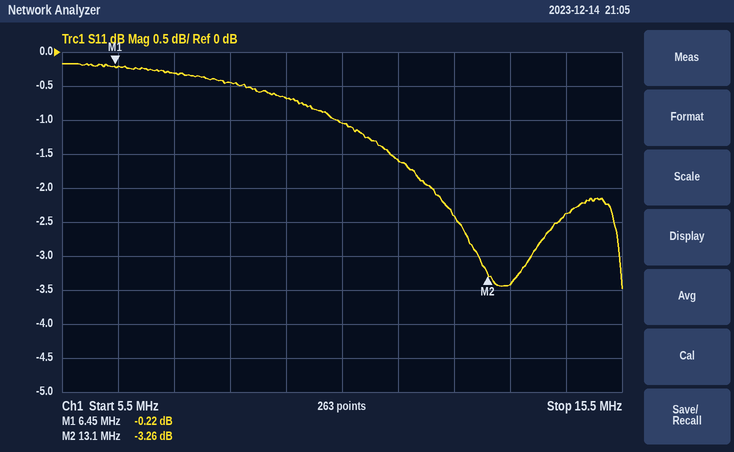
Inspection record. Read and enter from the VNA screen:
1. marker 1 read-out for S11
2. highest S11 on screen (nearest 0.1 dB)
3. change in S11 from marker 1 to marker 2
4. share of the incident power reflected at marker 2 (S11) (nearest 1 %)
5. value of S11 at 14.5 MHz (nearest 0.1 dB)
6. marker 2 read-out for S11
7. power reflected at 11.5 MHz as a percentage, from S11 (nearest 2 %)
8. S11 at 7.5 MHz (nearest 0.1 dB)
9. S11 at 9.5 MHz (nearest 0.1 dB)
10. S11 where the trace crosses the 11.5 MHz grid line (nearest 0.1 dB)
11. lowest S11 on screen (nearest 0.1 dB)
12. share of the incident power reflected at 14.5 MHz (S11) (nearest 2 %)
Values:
-0.22 dB
-0.2 dB
-3.04 dB
47 %
-2.4 dB
-3.26 dB
70 %
-0.3 dB
-0.7 dB
-1.6 dB
-3.5 dB
58 %
